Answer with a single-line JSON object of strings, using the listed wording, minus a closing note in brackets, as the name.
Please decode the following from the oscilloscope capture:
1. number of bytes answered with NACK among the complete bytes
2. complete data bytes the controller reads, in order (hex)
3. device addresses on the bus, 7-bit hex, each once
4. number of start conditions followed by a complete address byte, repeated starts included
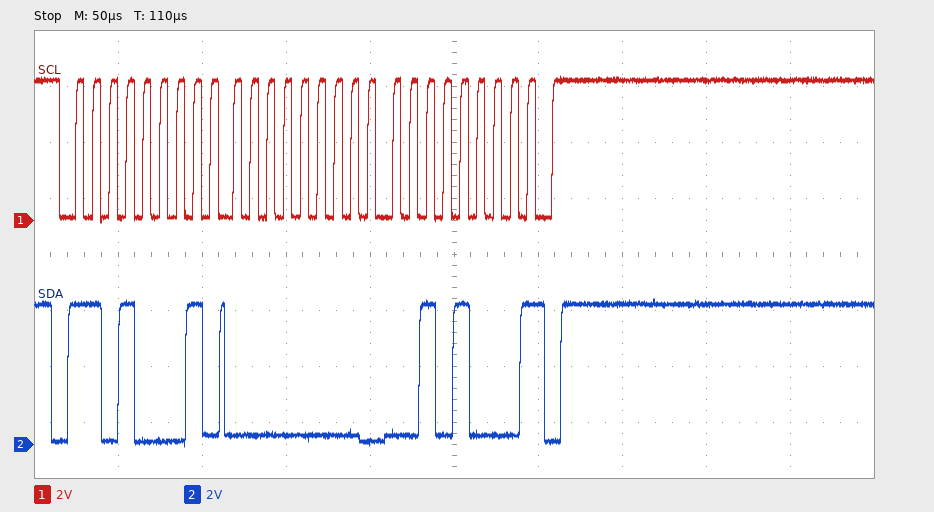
{"number of bytes answered with NACK among the complete bytes": "1", "complete data bytes the controller reads, in order": "00 28", "device addresses on the bus, 7-bit hex, each once": "0x68", "number of start conditions followed by a complete address byte, repeated starts included": "1"}
